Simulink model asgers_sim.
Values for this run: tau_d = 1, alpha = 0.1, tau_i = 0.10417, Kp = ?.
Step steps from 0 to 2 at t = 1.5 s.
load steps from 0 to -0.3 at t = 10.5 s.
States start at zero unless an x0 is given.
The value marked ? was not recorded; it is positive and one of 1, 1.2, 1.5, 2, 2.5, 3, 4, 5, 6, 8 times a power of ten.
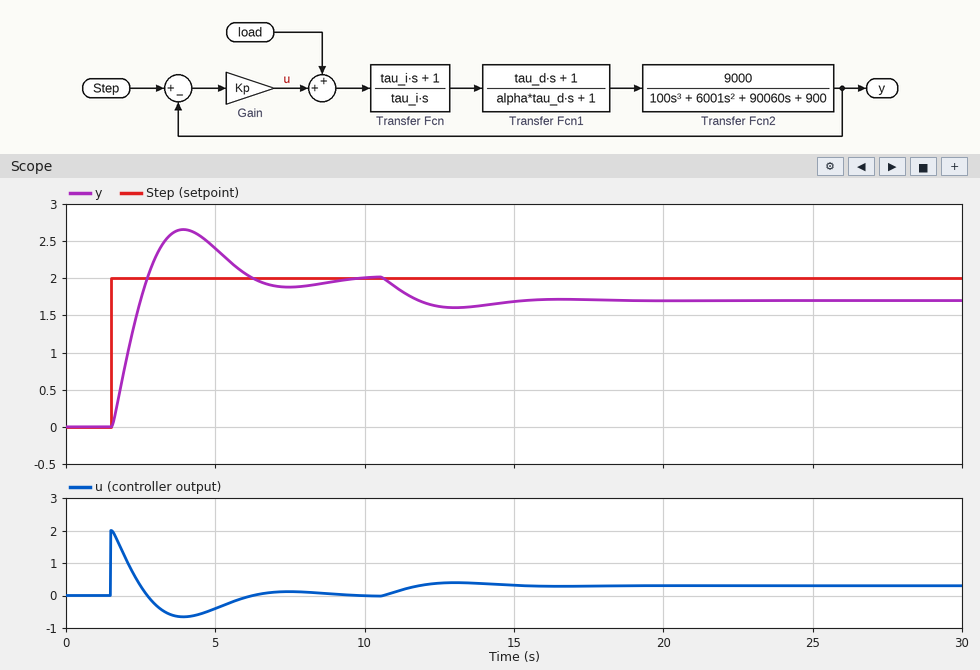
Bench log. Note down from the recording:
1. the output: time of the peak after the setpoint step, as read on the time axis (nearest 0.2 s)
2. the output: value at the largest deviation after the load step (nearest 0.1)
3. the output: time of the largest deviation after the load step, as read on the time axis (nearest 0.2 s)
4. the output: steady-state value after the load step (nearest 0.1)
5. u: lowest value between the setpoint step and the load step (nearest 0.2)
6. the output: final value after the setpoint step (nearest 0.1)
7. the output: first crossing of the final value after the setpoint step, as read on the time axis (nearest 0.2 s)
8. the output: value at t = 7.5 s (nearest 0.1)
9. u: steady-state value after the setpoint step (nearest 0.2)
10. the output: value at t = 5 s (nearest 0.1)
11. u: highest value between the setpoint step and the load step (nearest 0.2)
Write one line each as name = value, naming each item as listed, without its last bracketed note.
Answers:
the output: time of the peak after the setpoint step, as read on the time axis = 4.0 s
the output: value at the largest deviation after the load step = 1.6
the output: time of the largest deviation after the load step, as read on the time axis = 13.0 s
the output: steady-state value after the load step = 1.7
u: lowest value between the setpoint step and the load step = -0.6
the output: final value after the setpoint step = 2.0
the output: first crossing of the final value after the setpoint step, as read on the time axis = 2.8 s
the output: value at t = 7.5 s = 1.9
u: steady-state value after the setpoint step = 0.0
the output: value at t = 5 s = 2.4
u: highest value between the setpoint step and the load step = 2.0
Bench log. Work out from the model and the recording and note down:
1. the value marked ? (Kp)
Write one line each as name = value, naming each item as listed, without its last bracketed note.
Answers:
the value marked ? = 1
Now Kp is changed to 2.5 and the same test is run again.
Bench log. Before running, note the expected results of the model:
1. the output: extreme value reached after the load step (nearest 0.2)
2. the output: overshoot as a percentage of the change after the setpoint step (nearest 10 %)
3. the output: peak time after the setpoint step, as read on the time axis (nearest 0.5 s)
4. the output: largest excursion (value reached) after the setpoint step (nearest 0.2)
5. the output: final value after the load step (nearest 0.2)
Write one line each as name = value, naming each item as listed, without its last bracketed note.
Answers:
the output: extreme value reached after the load step = 1.8
the output: overshoot as a percentage of the change after the setpoint step = 20 %
the output: peak time after the setpoint step, as read on the time axis = 3.0 s
the output: largest excursion (value reached) after the setpoint step = 2.4
the output: final value after the load step = 1.8
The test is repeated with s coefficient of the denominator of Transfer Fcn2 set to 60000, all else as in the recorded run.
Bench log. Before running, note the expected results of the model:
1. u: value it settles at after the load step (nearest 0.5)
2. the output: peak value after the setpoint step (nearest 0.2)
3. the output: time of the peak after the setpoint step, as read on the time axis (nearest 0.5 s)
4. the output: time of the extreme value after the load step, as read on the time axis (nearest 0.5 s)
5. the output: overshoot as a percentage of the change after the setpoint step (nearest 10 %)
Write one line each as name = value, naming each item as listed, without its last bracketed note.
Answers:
u: value it settles at after the load step = 0.5
the output: peak value after the setpoint step = 2.6
the output: time of the peak after the setpoint step, as read on the time axis = 3.5 s
the output: time of the extreme value after the load step, as read on the time axis = 12.5 s
the output: overshoot as a percentage of the change after the setpoint step = 30 %
